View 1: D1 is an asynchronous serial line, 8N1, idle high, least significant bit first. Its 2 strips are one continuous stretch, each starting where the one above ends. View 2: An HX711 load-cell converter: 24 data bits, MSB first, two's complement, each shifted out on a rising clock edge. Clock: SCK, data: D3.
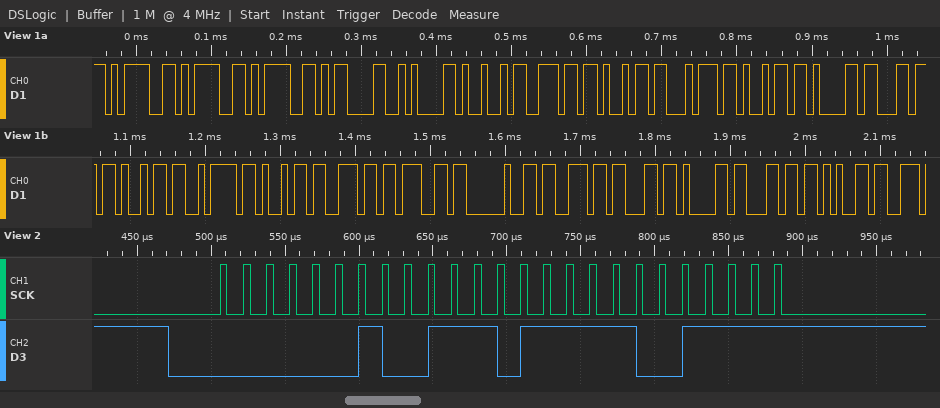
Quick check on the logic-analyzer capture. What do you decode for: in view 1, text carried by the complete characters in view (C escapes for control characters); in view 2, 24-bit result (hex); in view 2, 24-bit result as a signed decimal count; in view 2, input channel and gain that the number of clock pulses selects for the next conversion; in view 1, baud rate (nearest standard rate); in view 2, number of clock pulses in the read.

"===\r\nInitializing scale"
0x0277CF
161743
channel A, gain 128
115200 baud
25
